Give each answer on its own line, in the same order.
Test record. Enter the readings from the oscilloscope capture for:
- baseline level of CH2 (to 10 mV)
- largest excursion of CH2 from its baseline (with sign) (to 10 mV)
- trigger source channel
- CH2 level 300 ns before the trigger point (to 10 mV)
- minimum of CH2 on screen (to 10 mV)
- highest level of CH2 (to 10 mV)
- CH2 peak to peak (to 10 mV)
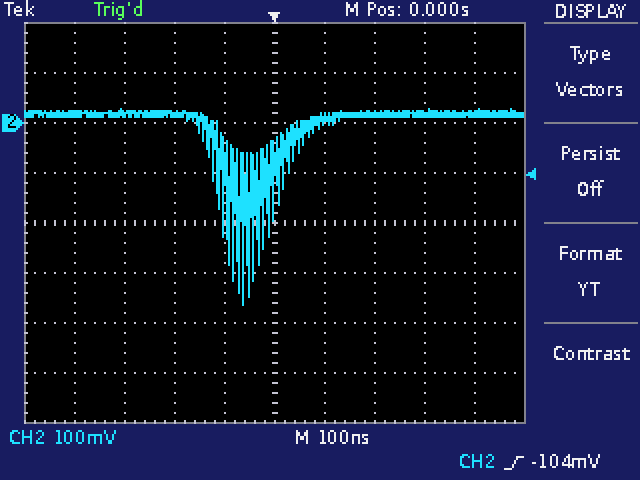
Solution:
20 mV
-380 mV
CH2
20 mV
-360 mV
30 mV
390 mV
